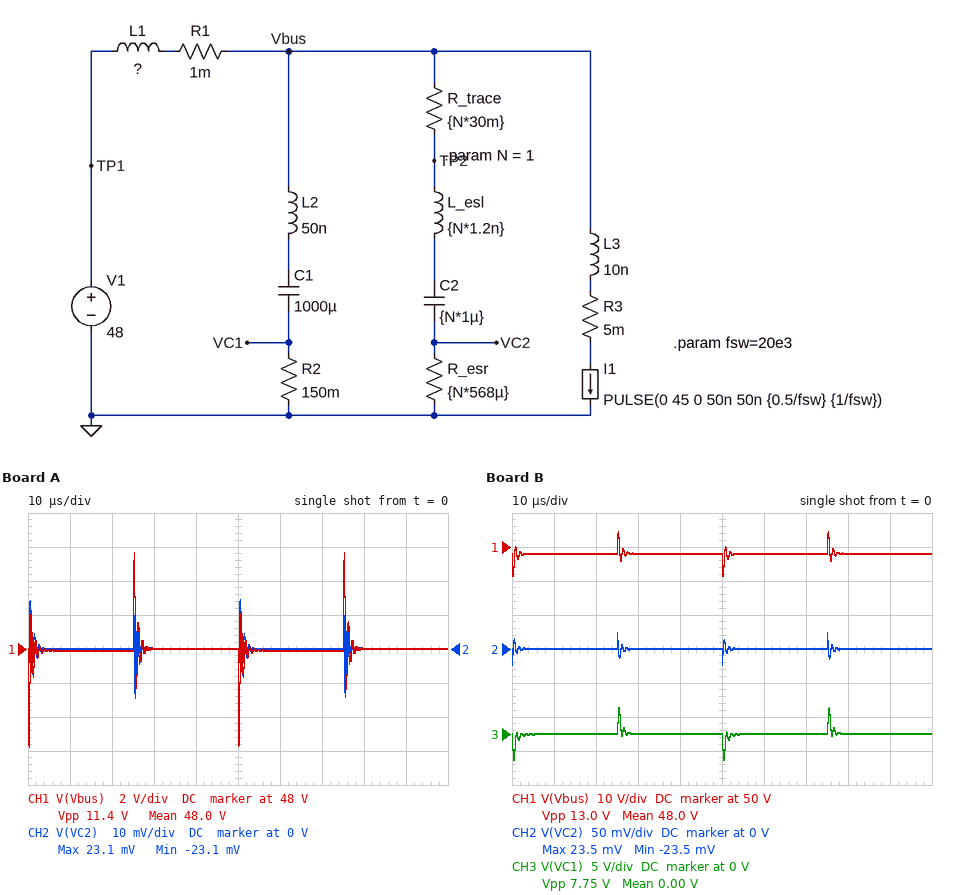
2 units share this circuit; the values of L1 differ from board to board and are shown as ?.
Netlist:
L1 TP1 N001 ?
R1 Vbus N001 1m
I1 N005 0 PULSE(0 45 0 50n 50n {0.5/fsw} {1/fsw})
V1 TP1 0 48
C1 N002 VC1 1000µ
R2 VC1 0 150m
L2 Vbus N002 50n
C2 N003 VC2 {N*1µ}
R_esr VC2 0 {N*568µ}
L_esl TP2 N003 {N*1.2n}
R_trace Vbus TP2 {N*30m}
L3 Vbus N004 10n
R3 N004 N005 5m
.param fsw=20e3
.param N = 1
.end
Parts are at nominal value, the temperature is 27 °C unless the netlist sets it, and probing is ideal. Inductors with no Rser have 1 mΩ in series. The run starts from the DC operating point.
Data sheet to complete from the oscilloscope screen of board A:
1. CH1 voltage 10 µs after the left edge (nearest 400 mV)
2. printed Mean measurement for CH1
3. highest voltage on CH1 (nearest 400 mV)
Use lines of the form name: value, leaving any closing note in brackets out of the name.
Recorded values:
CH1 voltage 10 µs after the left edge: 48.0 V
printed Mean measurement for CH1: 48.0 V
highest voltage on CH1: 53.6 V
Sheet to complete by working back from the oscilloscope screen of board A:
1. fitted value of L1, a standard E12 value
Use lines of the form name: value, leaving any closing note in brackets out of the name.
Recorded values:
fitted value of L1, a standard E12 value: 39 nH
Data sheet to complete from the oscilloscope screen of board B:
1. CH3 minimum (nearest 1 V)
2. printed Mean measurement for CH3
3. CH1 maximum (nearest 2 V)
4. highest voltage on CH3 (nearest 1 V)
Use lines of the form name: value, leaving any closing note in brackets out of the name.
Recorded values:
CH3 minimum: -4 V
printed Mean measurement for CH3: 0.00 V
CH1 maximum: 54 V
highest voltage on CH3: 4 V
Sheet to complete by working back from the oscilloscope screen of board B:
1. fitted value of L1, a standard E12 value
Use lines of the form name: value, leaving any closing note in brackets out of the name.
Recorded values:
fitted value of L1, a standard E12 value: 56 nH
